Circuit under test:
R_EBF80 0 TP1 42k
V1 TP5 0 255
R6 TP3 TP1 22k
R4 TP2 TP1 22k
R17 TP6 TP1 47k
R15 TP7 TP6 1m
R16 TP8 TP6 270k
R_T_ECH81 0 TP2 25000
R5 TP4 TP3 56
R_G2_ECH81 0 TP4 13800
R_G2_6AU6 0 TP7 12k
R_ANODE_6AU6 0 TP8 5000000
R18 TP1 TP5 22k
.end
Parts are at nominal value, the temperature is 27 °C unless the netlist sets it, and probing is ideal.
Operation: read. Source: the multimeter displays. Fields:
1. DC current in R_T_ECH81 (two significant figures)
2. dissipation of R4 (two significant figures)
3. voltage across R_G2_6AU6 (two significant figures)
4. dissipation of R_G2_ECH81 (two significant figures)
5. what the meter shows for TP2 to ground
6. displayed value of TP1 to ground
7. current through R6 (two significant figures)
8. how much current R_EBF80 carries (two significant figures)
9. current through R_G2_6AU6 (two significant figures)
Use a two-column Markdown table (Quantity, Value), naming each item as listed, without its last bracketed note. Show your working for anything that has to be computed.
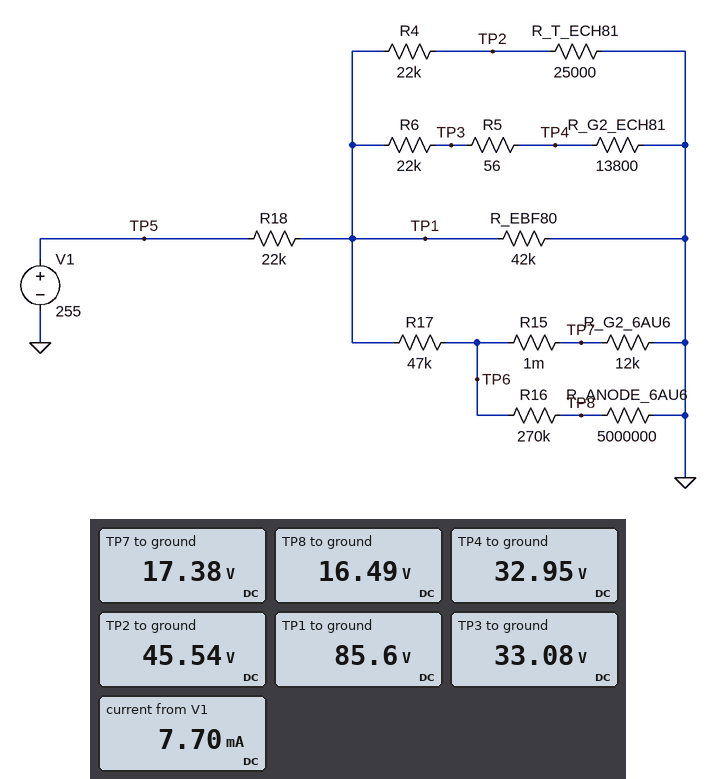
| Quantity | Value |
|---|---|
| DC current in R_T_ECH81 | (45.54 V) / 25 kΩ = 1.8 mA |
| dissipation of R4 | (85.6 V - 45.54 V)^2 / 22 kΩ = 73 mW |
| voltage across R_G2_6AU6 | 17.38 V = 17 V |
| dissipation of R_G2_ECH81 | (32.95 V)^2 / 13.8 kΩ = 79 mW |
| what the meter shows for TP2 to ground | 45.54 V |
| displayed value of TP1 to ground | 85.6 V |
| current through R6 | (85.6 V - 33.08 V) / 22 kΩ = 2.4 mA |
| how much current R_EBF80 carries | (85.6 V) / 42 kΩ = 2.0 mA |
| current through R_G2_6AU6 | (17.38 V) / 12 kΩ = 1.4 mA |
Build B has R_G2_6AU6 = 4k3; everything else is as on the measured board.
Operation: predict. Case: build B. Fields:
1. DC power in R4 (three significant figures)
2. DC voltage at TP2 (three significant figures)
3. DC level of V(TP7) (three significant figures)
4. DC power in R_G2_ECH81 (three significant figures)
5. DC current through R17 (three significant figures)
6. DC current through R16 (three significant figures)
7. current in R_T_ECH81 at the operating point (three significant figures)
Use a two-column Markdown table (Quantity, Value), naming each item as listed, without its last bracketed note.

| Quantity | Value |
|---|---|
| DC power in R4 | 70.3 mW |
| DC voltage at TP2 | 44.7 V |
| DC level of V(TP7) | 7.04 V |
| DC power in R_G2_ECH81 | 75.8 mW |
| DC current through R17 | 1.64 mA |
| DC current through R16 | 1.34 µA |
| current in R_T_ECH81 at the operating point | 1.79 mA |
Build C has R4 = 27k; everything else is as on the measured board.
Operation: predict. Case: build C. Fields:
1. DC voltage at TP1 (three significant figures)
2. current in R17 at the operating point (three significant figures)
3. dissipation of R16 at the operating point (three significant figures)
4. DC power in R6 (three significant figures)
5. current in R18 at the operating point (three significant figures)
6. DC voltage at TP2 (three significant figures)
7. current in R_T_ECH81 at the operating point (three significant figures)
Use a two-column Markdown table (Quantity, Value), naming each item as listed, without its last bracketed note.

| Quantity | Value |
|---|---|
| DC voltage at TP1 | 86.9 V |
| current in R17 at the operating point | 1.47 mA |
| dissipation of R16 at the operating point | 3.03 µW |
| DC power in R6 | 129 mW |
| current in R18 at the operating point | 7.64 mA |
| DC voltage at TP2 | 41.8 V |
| current in R_T_ECH81 at the operating point | 1.67 mA |
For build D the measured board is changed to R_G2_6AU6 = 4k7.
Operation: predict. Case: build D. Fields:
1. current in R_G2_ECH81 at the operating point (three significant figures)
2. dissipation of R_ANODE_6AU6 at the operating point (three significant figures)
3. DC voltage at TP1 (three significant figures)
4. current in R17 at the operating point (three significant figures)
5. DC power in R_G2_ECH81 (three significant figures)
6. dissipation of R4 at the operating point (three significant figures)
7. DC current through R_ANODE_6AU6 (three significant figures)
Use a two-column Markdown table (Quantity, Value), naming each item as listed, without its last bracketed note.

| Quantity | Value |
|---|---|
| current in R_G2_ECH81 at the operating point | 2.35 mA |
| dissipation of R_ANODE_6AU6 at the operating point | 10.5 µW |
| DC voltage at TP1 | 84.1 V |
| current in R17 at the operating point | 1.63 mA |
| DC power in R_G2_ECH81 | 76.0 mW |
| dissipation of R4 at the operating point | 70.5 mW |
| DC current through R_ANODE_6AU6 | 1.45 µA |
